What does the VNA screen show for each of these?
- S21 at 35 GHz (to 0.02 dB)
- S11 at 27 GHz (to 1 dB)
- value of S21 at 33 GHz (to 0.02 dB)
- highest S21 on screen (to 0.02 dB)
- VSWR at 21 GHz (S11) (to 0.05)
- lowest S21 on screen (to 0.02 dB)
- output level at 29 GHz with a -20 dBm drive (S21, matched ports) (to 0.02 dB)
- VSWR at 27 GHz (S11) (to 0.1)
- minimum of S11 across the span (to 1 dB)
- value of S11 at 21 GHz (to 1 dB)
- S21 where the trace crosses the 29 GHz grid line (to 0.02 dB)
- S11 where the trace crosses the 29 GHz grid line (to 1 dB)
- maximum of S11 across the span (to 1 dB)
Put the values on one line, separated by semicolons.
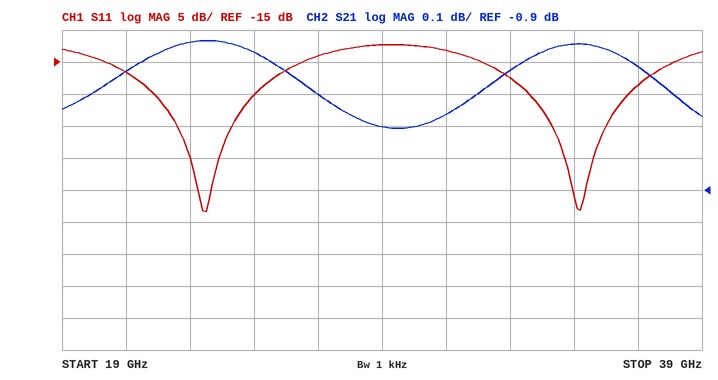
-0.44 dB; -14 dB; -0.52 dB; -0.44 dB; 1.35; -0.70 dB; -20.70 dBm; 1.5; -38 dB; -17 dB; -0.70 dB; -12 dB; -12 dB
